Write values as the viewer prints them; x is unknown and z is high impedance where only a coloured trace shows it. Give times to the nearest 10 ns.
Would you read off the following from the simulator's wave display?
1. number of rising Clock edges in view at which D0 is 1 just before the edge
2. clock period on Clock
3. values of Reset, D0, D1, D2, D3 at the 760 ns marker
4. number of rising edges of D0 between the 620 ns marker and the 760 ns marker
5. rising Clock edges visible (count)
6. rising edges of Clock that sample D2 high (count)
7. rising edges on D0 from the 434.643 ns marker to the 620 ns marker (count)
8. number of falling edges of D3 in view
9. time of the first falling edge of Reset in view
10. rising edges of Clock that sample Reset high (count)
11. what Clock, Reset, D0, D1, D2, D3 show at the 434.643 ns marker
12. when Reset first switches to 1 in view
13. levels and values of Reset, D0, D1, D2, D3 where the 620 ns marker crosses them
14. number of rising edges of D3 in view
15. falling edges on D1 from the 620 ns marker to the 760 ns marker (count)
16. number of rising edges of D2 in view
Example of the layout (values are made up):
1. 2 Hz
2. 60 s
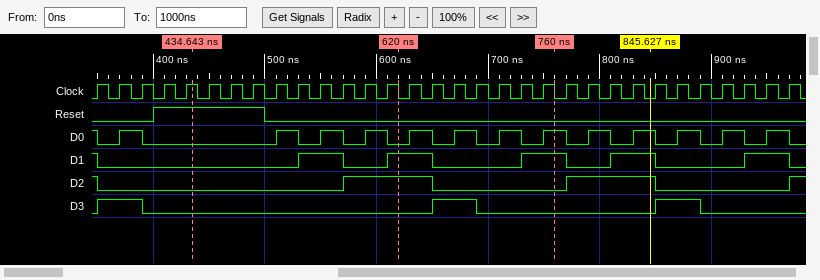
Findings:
1. 14
2. 20 ns
3. Reset=0, D0=1, D1=1, D2=0, D3=0
4. 4
5. 32
6. 9
7. 3
8. 3
9. 500 ns
10. 5
11. Clock=1, Reset=1, D0=0, D1=0, D2=0, D3=0
12. 400 ns
13. Reset=0, D0=0, D1=1, D2=1, D3=0
14. 3
15. 1
16. 3
